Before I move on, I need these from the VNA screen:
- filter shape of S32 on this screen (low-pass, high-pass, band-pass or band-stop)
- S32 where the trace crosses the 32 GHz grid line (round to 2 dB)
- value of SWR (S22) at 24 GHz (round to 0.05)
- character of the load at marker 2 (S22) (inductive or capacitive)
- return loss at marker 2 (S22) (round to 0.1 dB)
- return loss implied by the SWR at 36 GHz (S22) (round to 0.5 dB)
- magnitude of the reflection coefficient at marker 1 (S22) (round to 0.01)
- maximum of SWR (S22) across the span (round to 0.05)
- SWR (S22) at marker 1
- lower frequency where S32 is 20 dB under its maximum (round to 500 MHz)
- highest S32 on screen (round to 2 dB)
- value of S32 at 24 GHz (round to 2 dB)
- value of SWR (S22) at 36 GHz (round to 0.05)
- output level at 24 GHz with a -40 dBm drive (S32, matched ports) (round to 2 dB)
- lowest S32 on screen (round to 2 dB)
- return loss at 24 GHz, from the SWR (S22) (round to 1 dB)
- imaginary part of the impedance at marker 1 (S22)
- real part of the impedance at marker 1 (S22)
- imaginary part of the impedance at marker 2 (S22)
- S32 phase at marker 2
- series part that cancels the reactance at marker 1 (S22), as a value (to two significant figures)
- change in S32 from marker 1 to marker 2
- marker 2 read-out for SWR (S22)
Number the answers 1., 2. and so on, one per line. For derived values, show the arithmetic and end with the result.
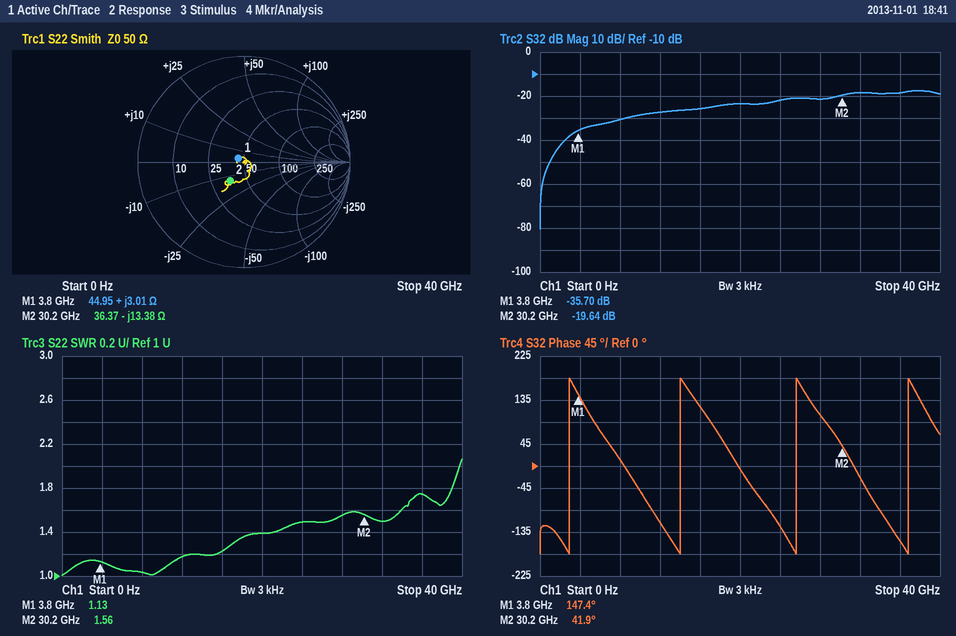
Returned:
1. high-pass
2. -18 dB
3. 1.50
4. capacitive
5. 13.2 dB
6. −20 log10((1.75 − 1)/(1.75 + 1)) ≈ 11.3 dB, so 11.5 dB to the nearest 0.5 dB
7. 0.06
8. 2.05
9. 1.13
10. 3.0 GHz
11. -18 dB
12. -22 dB
13. 1.75
14. -40 dBm + (-22 dB) = -62 dBm
15. -80 dB
16. −20 log10((1.5 − 1)/(1.5 + 1)) ≈ 14 dB
17. +3.01 Ω
18. 44.95 Ω
19. -13.38 Ω
20. 41.9°
21. C = 1/(2π × 3.8 GHz × 3.01 Ω) ≈ 14 pF
22. -19.64 − (-35.7) = 16.06 dB
23. 1.56
